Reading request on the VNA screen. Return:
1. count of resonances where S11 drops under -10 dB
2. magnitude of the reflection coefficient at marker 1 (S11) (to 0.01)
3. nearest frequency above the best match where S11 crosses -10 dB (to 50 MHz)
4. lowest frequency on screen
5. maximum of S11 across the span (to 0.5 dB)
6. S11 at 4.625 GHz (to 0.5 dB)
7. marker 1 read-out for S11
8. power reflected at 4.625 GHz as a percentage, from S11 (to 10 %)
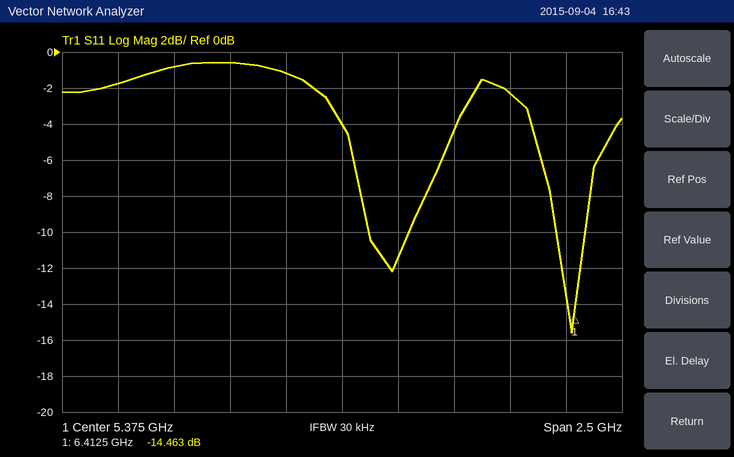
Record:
2
0.19
6.45 GHz
4.125 GHz
-0.5 dB
-1.0 dB
-14.463 dB
80 %
